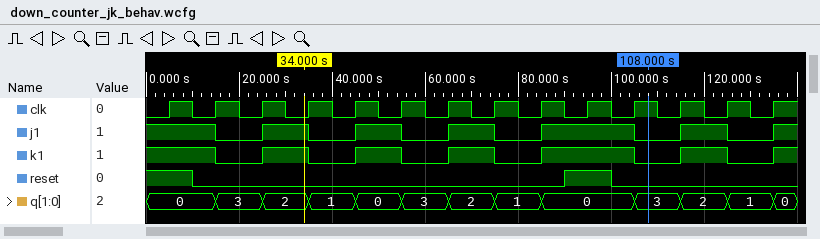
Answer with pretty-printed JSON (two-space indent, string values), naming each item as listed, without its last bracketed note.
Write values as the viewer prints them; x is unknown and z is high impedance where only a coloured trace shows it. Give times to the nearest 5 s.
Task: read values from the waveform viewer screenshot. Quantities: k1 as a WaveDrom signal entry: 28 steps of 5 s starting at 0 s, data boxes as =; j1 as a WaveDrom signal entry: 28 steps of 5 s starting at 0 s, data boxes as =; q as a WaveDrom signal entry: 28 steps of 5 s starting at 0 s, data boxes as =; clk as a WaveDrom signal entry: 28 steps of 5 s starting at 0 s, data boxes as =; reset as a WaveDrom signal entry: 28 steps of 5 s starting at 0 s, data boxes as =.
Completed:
{
  "k1 as a WaveDrom signal entry: 28 steps of 5 s starting at 0 s, data boxes as =": "{name: 'k1', wave: '1..0.1.0.1.0.1.0.1...0.1.0.1'}",
  "j1 as a WaveDrom signal entry: 28 steps of 5 s starting at 0 s, data boxes as =": "{name: 'j1', wave: '1..0.1.0.1.0.1.0.1...0.1.0.1'}",
  "q as a WaveDrom signal entry: 28 steps of 5 s starting at 0 s, data boxes as =": "{name: 'q', wave: '=..=.=.=.=.=.=.=.=...=.=.=.=', data: '0 3 2 1 0 3 2 1 0 3 2 1 0'}",
  "clk as a WaveDrom signal entry: 28 steps of 5 s starting at 0 s, data boxes as =": "{name: 'clk', wave: '0101010101010101010101010101'}",
  "reset as a WaveDrom signal entry: 28 steps of 5 s starting at 0 s, data boxes as =": "{name: 'reset', wave: '1.0...............1.0.......'}"
}
